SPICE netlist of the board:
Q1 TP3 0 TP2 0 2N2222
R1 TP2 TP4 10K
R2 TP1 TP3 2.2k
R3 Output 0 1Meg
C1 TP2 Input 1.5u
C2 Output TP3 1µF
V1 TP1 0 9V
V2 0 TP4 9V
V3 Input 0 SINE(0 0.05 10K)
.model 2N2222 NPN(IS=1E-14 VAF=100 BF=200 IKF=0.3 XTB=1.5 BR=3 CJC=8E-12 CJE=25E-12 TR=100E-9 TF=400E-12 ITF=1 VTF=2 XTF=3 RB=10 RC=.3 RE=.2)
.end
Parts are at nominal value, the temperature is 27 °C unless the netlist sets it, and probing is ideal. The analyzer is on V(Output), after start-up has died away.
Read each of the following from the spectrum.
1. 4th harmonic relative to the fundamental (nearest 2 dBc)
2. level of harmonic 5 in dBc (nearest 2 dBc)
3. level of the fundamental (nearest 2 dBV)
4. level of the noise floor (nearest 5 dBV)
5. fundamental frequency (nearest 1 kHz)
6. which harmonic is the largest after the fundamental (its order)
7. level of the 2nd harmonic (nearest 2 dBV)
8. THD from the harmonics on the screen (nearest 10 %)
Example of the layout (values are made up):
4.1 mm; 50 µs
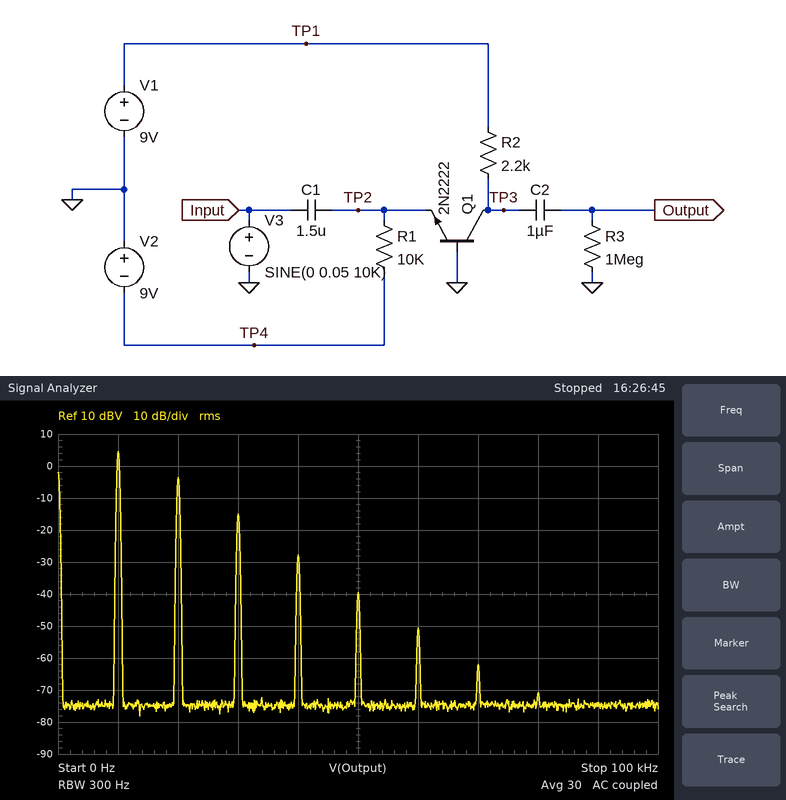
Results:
-32 dBc; -44 dBc; 4 dBV; -75 dBV; 10 kHz; 2; -4 dBV; 40 %
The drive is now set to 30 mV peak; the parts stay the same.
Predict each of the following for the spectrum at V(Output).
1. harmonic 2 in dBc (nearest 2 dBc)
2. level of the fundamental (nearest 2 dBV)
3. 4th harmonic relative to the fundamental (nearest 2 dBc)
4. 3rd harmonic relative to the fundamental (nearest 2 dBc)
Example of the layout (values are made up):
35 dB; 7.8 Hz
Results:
-12 dBc; 2 dBV; -44 dBc; -28 dBc
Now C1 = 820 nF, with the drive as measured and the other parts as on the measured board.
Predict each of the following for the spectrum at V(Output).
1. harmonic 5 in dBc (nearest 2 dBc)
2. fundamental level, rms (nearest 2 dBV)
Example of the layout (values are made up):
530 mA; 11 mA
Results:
-42 dBc; 4 dBV
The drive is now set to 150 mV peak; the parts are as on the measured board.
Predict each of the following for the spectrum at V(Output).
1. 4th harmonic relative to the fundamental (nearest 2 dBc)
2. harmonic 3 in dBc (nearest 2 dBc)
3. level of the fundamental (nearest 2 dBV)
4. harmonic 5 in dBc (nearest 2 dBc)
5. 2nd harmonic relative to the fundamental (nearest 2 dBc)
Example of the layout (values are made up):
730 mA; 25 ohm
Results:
-14 dBc; -8 dBc; 8 dBV; -22 dBc; -2 dBc
